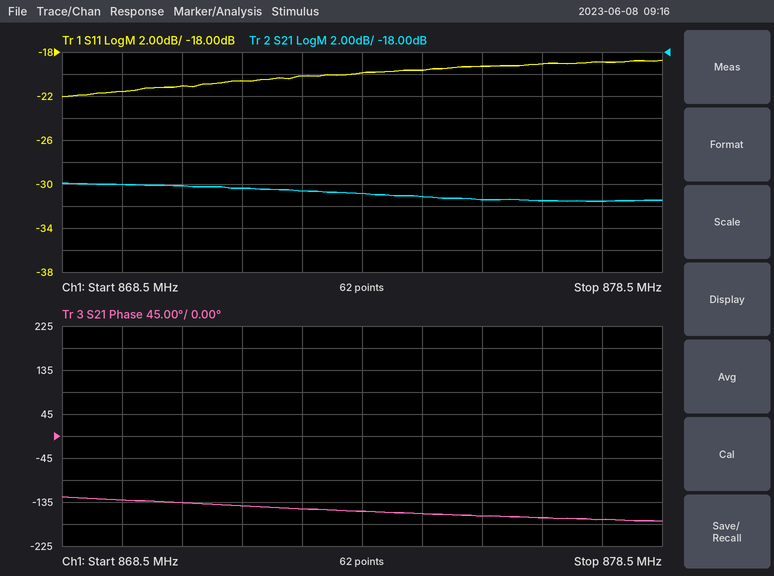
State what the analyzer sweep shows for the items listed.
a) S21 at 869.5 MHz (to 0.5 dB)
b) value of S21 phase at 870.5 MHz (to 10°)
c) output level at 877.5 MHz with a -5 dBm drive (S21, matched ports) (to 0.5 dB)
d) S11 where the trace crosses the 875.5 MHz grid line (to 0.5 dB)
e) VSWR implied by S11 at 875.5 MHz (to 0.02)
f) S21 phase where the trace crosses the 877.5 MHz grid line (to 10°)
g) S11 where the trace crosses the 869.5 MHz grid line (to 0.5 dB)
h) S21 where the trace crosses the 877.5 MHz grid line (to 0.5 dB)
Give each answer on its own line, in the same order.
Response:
-30.0 dB
-140°
-36.5 dBm
-19.5 dB
1.24
-170°
-21.5 dB
-31.5 dB
